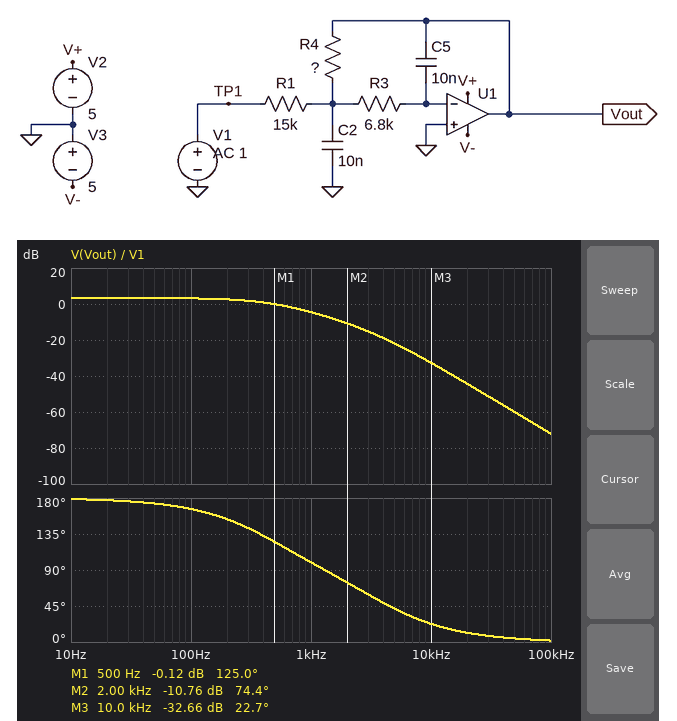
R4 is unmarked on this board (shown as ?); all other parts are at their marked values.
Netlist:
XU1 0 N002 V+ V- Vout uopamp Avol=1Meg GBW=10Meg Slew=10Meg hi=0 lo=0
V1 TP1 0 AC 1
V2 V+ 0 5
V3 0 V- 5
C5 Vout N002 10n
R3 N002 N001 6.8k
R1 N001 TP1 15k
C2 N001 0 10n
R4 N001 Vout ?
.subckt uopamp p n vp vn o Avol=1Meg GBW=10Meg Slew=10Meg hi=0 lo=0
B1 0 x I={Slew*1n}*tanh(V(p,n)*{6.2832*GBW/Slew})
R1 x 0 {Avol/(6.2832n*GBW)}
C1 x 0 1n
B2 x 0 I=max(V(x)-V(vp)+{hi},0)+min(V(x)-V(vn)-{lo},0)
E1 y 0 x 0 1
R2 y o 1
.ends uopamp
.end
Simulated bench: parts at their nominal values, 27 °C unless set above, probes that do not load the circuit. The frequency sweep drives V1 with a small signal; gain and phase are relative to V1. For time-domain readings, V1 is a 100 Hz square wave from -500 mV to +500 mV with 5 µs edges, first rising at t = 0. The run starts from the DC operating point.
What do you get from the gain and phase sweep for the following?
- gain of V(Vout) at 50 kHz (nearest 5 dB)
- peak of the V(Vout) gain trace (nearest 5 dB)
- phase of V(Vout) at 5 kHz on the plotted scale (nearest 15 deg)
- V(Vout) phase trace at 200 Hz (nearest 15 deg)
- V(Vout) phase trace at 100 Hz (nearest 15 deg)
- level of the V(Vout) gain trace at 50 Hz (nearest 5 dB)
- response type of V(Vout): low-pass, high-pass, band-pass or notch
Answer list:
-60 dB
5 dB
45 deg
150 deg
165 deg
5 dB
low-pass
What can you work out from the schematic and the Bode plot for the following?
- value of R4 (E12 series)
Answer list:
22 kΩ
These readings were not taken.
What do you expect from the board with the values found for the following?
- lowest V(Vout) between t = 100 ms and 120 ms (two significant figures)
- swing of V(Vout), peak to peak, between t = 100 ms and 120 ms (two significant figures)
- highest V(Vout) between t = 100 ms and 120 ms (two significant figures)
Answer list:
-730 mV
1.5 V
730 mV
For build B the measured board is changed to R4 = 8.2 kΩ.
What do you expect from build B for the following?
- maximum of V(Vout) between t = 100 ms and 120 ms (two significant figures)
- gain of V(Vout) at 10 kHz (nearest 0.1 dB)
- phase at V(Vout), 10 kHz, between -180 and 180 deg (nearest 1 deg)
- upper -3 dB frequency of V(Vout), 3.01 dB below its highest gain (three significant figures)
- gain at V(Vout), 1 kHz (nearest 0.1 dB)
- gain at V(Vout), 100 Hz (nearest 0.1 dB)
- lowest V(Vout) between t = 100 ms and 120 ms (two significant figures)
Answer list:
270 mV
-32.9 dB
29 deg
1.00 kHz
-8.2 dB
-5.3 dB
-270 mV
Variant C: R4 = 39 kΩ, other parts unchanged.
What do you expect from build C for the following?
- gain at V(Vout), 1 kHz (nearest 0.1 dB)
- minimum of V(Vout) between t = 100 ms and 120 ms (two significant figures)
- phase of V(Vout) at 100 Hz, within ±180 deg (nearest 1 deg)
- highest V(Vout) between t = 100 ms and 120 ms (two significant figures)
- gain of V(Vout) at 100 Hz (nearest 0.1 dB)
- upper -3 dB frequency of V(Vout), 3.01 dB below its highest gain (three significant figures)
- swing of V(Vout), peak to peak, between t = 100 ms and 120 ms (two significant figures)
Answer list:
-3.7 dB
-1.3 V
158 deg
1.3 V
7.7 dB
268 Hz
2.6 V
